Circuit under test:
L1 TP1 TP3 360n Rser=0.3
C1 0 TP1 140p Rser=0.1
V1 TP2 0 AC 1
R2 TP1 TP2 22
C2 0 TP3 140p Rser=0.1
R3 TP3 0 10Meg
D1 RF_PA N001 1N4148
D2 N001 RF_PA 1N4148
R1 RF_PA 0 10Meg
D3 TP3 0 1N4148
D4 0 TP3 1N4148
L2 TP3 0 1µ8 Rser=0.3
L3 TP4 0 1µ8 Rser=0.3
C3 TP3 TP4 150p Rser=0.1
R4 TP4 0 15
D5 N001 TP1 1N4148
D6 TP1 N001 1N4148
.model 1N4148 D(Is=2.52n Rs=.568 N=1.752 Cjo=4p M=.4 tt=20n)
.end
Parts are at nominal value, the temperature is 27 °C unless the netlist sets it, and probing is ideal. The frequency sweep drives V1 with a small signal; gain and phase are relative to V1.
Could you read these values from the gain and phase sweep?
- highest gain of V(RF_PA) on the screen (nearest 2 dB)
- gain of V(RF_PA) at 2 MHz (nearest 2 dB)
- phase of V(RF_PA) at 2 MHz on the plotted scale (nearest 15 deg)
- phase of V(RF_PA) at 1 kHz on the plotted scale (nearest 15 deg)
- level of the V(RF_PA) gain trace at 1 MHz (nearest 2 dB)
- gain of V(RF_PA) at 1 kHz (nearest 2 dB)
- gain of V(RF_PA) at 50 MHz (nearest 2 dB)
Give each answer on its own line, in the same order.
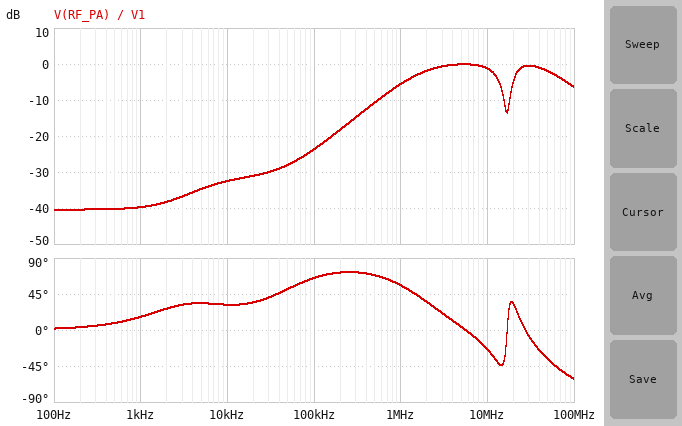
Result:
0 dB
-2 dB
30 deg
15 deg
-6 dB
-40 dB
-2 dB
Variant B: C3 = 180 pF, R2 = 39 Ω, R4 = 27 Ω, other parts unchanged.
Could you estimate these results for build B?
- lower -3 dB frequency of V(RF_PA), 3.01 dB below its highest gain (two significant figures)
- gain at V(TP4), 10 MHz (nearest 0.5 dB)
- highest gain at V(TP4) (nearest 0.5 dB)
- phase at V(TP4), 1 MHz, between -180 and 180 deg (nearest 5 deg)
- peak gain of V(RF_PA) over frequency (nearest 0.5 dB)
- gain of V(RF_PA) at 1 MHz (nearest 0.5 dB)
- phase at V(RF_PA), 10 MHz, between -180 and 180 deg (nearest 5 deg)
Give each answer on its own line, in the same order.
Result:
2.3 MHz
-11.5 dB
-8.5 dB
-135 deg
-0.5 dB
-9.5 dB
-35 deg
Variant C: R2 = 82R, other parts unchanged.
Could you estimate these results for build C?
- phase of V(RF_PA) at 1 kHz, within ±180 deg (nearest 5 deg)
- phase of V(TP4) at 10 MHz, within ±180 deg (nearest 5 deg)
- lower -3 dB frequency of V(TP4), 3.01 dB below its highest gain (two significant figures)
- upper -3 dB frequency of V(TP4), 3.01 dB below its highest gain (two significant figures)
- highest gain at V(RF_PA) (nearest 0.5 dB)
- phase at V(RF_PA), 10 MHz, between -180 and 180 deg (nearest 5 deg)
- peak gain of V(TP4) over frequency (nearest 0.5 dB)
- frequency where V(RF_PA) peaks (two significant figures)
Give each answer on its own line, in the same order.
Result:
15 deg
30 deg
19 MHz
31 MHz
-0.5 dB
-55 deg
-15.5 dB
5.5 MHz
